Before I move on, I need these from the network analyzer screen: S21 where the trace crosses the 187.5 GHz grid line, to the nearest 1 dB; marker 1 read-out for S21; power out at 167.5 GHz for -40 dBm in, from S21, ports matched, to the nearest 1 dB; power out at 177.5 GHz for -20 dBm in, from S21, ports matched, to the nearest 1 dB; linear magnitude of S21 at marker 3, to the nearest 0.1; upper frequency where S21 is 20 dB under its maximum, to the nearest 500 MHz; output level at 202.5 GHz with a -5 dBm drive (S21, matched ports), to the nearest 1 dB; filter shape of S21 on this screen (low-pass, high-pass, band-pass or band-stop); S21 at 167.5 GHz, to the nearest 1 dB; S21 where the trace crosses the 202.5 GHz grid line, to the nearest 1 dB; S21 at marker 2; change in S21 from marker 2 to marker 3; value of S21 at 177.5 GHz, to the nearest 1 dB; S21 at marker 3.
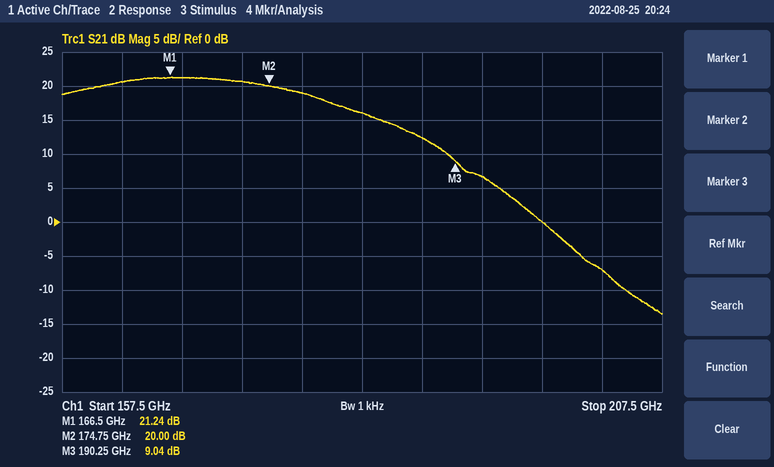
12 dB
21.24 dB
-19 dBm
-1 dBm
2.8
196.5 GHz
-12 dBm
low-pass
21 dB
-7 dB
20.00 dB
-10.96 dB
19 dB
9.04 dB
